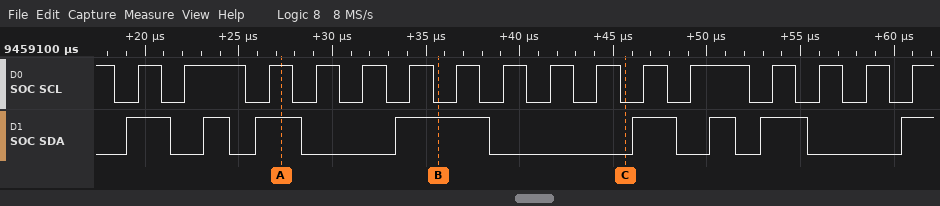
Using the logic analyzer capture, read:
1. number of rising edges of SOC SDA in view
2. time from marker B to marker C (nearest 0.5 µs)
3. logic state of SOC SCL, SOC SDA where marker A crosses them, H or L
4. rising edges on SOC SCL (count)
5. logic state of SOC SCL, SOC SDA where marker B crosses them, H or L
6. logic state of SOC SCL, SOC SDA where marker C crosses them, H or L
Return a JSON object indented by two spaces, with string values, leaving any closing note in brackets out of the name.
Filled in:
{
  "number of rising edges of SOC SDA in view": "8",
  "time from marker B to marker C": "10 µs",
  "logic state of SOC SCL, SOC SDA where marker A crosses them, H or L": "SOC SCL=H, SOC SDA=H",
  "rising edges on SOC SCL": "16",
  "logic state of SOC SCL, SOC SDA where marker B crosses them, H or L": "SOC SCL=L, SOC SDA=H",
  "logic state of SOC SCL, SOC SDA where marker C crosses them, H or L": "SOC SCL=L, SOC SDA=L"
}
